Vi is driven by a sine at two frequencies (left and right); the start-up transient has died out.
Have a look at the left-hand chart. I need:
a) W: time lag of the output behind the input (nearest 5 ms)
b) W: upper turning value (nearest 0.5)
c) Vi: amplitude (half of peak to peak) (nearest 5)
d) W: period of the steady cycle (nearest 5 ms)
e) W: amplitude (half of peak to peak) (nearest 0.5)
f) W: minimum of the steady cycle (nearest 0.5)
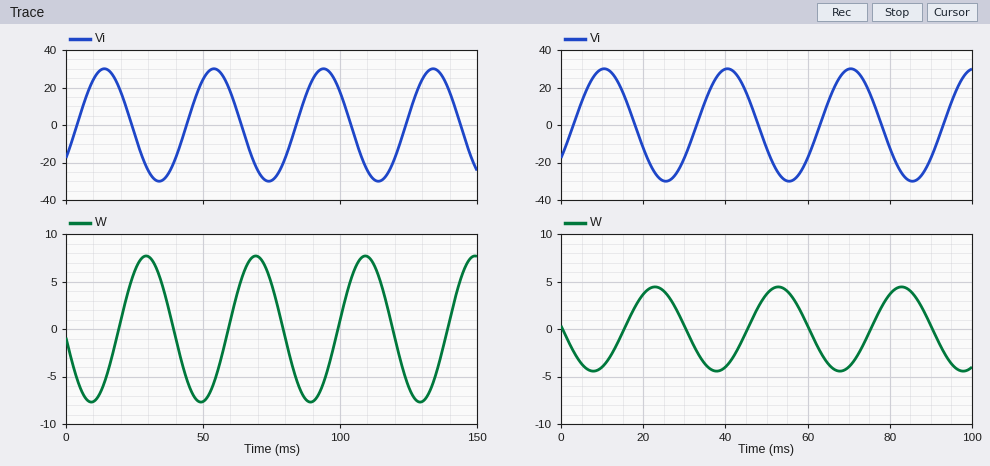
15 ms
7.5
30
40 ms
7.5
-7.5
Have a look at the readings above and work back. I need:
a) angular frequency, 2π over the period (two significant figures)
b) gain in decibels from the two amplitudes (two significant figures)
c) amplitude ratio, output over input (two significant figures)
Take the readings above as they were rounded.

0.16 rad/ms
-12 dB
0.25
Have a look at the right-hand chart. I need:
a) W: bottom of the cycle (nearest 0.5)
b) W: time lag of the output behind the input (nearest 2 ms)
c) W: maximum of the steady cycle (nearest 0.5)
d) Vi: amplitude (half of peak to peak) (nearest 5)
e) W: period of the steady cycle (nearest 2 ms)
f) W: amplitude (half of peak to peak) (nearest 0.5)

-4.5
12 ms
4.5
30
30 ms
4.5
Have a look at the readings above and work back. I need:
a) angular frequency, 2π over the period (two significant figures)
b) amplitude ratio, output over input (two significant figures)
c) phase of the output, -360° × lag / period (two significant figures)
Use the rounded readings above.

0.21 rad/ms
0.15
-140°
